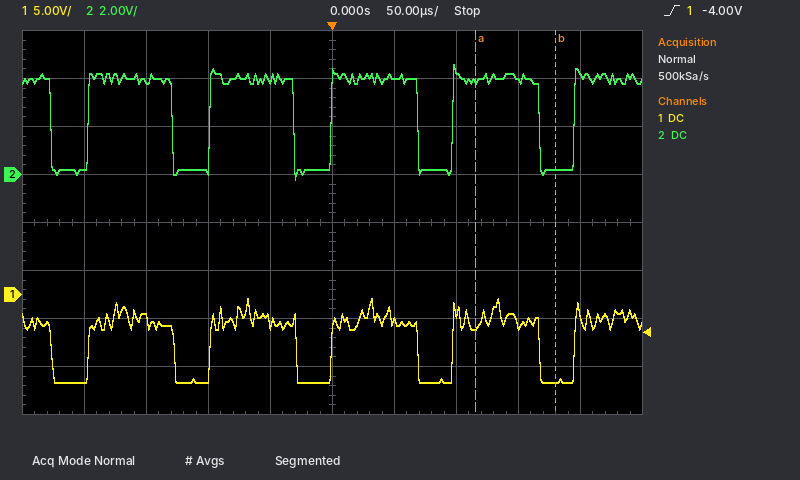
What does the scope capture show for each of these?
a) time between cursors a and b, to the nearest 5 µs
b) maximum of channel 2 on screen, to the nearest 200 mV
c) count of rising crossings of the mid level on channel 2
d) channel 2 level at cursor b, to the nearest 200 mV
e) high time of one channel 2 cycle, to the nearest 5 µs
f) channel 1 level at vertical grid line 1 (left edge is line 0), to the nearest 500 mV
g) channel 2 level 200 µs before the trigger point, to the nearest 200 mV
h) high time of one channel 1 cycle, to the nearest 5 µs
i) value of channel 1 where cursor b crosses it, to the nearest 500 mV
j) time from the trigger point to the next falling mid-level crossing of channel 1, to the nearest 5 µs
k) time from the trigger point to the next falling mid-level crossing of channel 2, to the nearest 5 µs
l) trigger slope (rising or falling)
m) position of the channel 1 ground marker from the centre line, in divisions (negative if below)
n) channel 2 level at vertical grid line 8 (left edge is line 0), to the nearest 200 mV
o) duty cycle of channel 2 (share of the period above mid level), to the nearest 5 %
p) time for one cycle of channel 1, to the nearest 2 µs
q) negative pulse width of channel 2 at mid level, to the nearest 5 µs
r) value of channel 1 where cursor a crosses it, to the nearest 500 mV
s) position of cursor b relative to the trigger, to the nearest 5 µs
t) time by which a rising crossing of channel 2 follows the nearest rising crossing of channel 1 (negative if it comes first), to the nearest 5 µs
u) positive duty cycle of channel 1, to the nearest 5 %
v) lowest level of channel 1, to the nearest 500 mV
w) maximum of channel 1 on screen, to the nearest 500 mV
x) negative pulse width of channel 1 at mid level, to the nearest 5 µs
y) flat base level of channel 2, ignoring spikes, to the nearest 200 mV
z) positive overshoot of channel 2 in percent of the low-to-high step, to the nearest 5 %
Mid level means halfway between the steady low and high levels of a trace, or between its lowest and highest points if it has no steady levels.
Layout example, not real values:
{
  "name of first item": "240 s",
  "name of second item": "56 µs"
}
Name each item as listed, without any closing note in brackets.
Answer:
{
  "time between cursors a and b, to the nearest 5 µs": "65 µs",
  "maximum of channel 2 on screen, to the nearest 200 mV": "4.6 V",
  "count of rising crossings of the mid level on channel 2": "5",
  "channel 2 level at cursor b, to the nearest 200 mV": "200 mV",
  "high time of one channel 2 cycle, to the nearest 5 µs": "70 µs",
  "channel 1 level at vertical grid line 1 (left edge is line 0), to the nearest 500 mV": "-9.0 V",
  "channel 2 level 200 µs before the trigger point, to the nearest 200 mV": "400 mV",
  "high time of one channel 1 cycle, to the nearest 5 µs": "70 µs",
  "value of channel 1 where cursor b crosses it, to the nearest 500 mV": "-9.0 V",
  "time from the trigger point to the next falling mid-level crossing of channel 1, to the nearest 5 µs": "70 µs",
  "time from the trigger point to the next falling mid-level crossing of channel 2, to the nearest 5 µs": "70 µs",
  "trigger slope": "rising",
  "position of the channel 1 ground marker from the centre line, in divisions": "-1.5 div",
  "channel 2 level at vertical grid line 8 (left edge is line 0), to the nearest 200 mV": "4.0 V",
  "duty cycle of channel 2 (share of the period above mid level), to the nearest 5 %": "70 %",
  "time for one cycle of channel 1, to the nearest 2 µs": "98 µs",
  "negative pulse width of channel 2 at mid level, to the nearest 5 µs": "30 µs",
  "value of channel 1 where cursor a crosses it, to the nearest 500 mV": "-3.5 V",
  "position of cursor b relative to the trigger, to the nearest 5 µs": "+180 µs",
  "time by which a rising crossing of channel 2 follows the nearest rising crossing of channel 1 (negative if it comes first), to the nearest 5 µs": "0 µs",
  "positive duty cycle of channel 1, to the nearest 5 %": "70 %",
  "lowest level of channel 1, to the nearest 500 mV": "-9.0 V",
  "maximum of channel 1 on screen, to the nearest 500 mV": "-500 mV",
  "negative pulse width of channel 1 at mid level, to the nearest 5 µs": "30 µs",
  "flat base level of channel 2, ignoring spikes, to the nearest 200 mV": "200 mV",
  "positive overshoot of channel 2 in percent of the low-to-high step, to the nearest 5 %": "15 %"
}
